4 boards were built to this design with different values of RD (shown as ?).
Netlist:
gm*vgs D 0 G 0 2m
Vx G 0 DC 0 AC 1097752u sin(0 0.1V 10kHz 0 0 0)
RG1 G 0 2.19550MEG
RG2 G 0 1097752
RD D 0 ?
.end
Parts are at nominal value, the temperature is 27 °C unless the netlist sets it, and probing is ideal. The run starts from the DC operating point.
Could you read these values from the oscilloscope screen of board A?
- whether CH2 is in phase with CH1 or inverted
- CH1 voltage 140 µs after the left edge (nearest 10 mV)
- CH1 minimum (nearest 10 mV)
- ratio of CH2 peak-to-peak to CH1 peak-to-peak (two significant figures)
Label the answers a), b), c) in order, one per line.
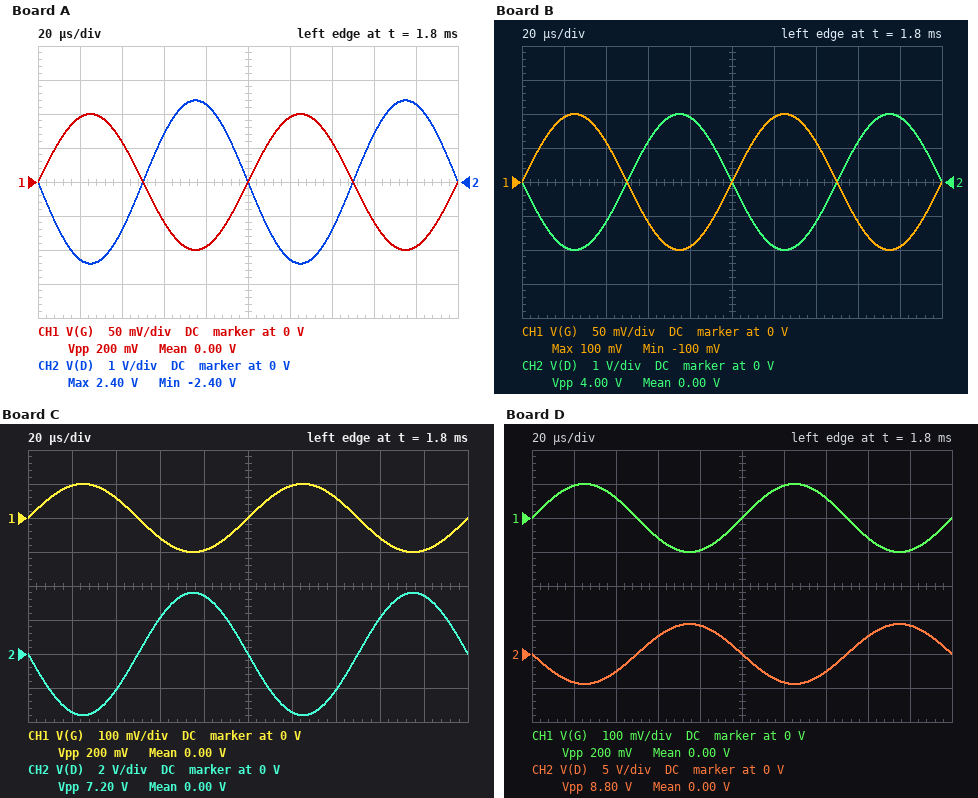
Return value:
a) inverted
b) 60 mV
c) -100 mV
d) 24
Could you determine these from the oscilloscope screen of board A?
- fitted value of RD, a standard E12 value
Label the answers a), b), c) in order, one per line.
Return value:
a) 12 kΩ
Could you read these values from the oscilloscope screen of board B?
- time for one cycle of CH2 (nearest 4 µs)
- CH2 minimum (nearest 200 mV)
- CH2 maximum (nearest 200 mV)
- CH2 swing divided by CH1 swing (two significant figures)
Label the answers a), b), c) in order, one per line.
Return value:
a) 100 µs
b) -2.0 V
c) 2.0 V
d) 20
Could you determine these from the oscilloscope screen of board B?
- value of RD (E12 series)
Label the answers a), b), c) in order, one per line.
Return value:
a) 10 kΩ
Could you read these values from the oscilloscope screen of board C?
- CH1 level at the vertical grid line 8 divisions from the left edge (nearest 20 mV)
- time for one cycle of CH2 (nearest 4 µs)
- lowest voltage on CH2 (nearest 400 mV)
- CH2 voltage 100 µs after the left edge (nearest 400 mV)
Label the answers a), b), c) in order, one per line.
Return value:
a) -60 mV
b) 100 µs
c) -3.6 V
d) 0 V
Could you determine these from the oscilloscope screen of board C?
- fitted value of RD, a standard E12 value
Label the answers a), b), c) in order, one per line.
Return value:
a) 18 kΩ
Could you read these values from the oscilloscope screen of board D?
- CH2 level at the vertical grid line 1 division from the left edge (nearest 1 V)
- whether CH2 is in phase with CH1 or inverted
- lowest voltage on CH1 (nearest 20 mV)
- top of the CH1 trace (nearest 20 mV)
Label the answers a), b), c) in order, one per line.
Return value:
a) -4 V
b) inverted
c) -100 mV
d) 100 mV
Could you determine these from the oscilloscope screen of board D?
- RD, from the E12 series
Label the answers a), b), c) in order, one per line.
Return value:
a) 22 kΩ
